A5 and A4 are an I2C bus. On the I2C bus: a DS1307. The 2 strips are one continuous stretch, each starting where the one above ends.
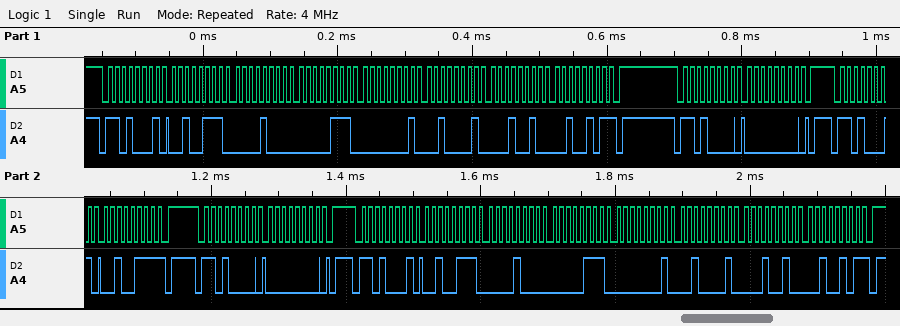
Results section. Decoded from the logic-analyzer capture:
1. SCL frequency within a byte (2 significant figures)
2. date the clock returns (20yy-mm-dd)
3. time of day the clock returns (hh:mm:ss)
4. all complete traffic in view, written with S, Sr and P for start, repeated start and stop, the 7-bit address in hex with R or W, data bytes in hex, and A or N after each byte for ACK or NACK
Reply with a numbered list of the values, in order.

1. 100 kHz
2. 2025-12-21
3. 07:08:27
4. S 68R A 27 A 08 A 07 A 01 A 21 A 12 A 25 N P S 68W A 00 A P S 68R A 27 N P S 68W A 00 A P S 68R A 27 A 08 A 07 A 01 A 21 A 12 A 25 N P
